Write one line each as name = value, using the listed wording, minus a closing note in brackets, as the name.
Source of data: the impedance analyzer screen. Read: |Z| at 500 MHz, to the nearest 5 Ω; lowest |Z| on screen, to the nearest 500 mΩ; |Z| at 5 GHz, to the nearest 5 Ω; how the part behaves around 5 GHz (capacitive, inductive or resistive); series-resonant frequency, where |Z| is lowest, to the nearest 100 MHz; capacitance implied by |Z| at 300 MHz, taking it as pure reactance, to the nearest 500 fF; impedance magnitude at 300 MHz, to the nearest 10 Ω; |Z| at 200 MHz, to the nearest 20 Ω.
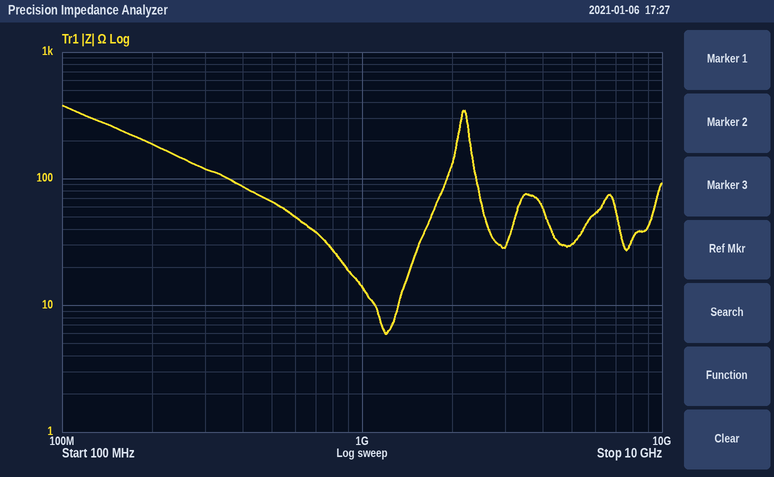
|Z| at 500 MHz, to the nearest 5 Ω = 65 Ω
lowest |Z| on screen, to the nearest 500 mΩ = 6.0 Ω
|Z| at 5 GHz, to the nearest 5 Ω = 30 Ω
how the part behaves around 5 GHz = resistive
series-resonant frequency, where |Z| is lowest, to the nearest 100 MHz = 1.2 GHz
capacitance implied by |Z| at 300 MHz, taking it as pure reactance, to the nearest 500 fF = 4.5 pF
impedance magnitude at 300 MHz, to the nearest 10 Ω = 120 Ω
|Z| at 200 MHz, to the nearest 20 Ω = 180 Ω
